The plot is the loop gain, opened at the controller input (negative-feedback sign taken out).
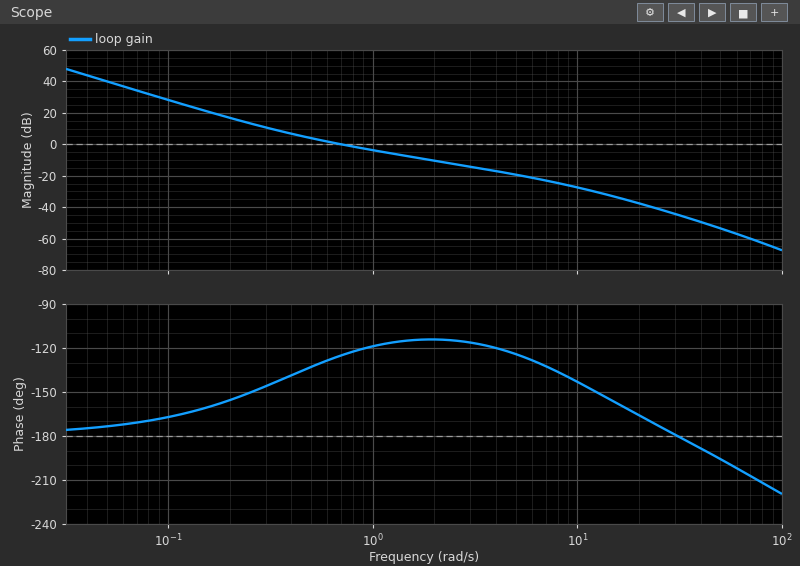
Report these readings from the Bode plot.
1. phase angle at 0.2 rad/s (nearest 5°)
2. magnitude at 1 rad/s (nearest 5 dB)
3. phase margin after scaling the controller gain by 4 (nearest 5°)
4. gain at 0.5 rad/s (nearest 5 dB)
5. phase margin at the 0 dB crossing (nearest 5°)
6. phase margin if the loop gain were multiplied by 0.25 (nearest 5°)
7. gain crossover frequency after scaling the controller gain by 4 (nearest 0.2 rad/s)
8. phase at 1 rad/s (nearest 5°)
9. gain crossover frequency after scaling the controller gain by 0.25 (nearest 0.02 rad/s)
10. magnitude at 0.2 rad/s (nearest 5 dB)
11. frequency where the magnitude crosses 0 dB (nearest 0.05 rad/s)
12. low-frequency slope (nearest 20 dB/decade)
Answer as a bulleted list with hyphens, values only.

- -155°
- -5 dB
- 65°
- 5 dB
- 55°
- 30°
- 2.4 rad/s
- -120°
- 0.28 rad/s
- 15 dB
- 0.70 rad/s
- -40 dB/decade
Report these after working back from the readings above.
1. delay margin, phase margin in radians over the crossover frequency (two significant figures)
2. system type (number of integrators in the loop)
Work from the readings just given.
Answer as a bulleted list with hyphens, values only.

- 1.4 s
- 2
